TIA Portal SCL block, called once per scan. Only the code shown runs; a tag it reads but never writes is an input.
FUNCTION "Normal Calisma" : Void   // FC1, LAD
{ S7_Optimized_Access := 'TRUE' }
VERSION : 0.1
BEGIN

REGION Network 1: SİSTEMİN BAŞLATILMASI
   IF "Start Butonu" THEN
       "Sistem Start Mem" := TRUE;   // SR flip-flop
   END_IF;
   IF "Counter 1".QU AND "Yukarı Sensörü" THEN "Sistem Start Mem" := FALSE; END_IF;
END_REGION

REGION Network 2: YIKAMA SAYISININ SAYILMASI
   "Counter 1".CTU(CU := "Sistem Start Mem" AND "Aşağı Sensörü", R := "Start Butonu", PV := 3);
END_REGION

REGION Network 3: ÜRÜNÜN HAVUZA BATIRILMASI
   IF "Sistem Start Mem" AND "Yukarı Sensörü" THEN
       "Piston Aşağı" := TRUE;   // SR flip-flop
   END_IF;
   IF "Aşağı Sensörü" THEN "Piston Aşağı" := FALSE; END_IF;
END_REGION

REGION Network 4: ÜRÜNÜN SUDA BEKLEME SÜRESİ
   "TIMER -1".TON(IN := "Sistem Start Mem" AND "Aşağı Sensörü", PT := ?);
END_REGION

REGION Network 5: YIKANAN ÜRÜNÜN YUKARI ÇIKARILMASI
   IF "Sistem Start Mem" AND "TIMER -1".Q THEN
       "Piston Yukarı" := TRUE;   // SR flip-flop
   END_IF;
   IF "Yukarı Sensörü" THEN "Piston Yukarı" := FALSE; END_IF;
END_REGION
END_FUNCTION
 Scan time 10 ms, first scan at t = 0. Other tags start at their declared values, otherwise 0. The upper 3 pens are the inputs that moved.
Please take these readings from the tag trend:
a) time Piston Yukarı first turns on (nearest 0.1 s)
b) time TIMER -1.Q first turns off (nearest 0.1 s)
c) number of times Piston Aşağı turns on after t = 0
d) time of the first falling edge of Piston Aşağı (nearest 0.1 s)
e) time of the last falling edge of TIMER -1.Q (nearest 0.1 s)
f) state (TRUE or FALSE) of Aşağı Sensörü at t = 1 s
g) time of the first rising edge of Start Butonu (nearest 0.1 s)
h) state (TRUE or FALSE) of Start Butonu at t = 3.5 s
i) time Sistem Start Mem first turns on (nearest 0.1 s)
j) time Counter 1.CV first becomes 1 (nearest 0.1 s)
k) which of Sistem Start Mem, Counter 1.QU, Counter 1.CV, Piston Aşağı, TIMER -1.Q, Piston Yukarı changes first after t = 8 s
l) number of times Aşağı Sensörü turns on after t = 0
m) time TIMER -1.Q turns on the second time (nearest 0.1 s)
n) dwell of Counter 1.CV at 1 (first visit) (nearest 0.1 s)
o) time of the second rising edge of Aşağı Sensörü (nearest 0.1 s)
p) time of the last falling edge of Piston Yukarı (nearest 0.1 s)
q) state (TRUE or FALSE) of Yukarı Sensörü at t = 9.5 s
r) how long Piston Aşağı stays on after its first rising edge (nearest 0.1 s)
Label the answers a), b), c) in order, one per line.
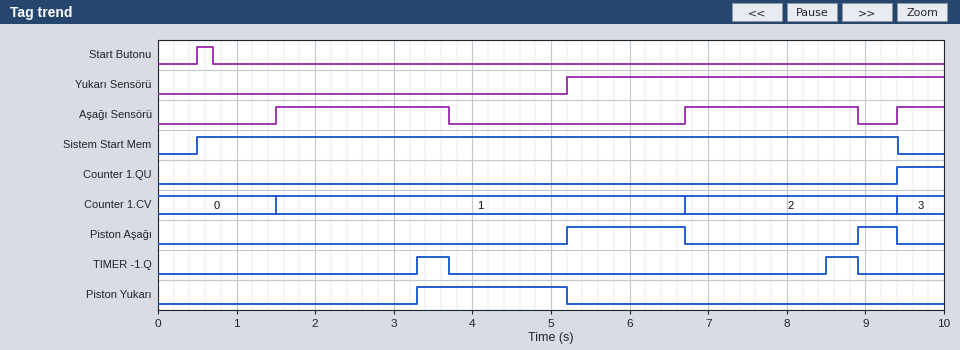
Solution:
a) 3.3 s
b) 3.7 s
c) 2
d) 6.7 s
e) 8.9 s
f) FALSE
g) 0.5 s
h) FALSE
i) 0.5 s
j) 1.5 s
k) TIMER -1.Q
l) 3
m) 8.5 s
n) 5.2 s
o) 6.7 s
p) 5.2 s
q) TRUE
r) 1.5 s
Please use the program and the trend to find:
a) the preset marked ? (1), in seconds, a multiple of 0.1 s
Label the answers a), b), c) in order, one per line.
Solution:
a) 1.8 s
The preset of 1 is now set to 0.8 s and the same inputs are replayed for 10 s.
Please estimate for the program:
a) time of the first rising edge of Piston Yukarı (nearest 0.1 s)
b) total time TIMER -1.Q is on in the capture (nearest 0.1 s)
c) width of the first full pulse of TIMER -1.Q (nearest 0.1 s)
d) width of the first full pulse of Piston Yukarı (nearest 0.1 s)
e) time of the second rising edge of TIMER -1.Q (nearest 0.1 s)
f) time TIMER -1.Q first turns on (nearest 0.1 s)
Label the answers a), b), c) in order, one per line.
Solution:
a) 2.3 s
b) 2.8 s
c) 1.4 s
d) 2.9 s
e) 7.5 s
f) 2.3 s
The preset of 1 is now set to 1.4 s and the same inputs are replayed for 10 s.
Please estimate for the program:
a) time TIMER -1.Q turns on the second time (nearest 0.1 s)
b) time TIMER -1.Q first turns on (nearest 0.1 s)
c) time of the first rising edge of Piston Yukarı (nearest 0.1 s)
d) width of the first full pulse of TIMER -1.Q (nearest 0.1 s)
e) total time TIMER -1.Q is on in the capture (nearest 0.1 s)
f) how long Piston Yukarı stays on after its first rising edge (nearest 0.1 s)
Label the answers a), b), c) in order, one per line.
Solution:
a) 8.1 s
b) 2.9 s
c) 2.9 s
d) 0.8 s
e) 1.6 s
f) 2.3 s
